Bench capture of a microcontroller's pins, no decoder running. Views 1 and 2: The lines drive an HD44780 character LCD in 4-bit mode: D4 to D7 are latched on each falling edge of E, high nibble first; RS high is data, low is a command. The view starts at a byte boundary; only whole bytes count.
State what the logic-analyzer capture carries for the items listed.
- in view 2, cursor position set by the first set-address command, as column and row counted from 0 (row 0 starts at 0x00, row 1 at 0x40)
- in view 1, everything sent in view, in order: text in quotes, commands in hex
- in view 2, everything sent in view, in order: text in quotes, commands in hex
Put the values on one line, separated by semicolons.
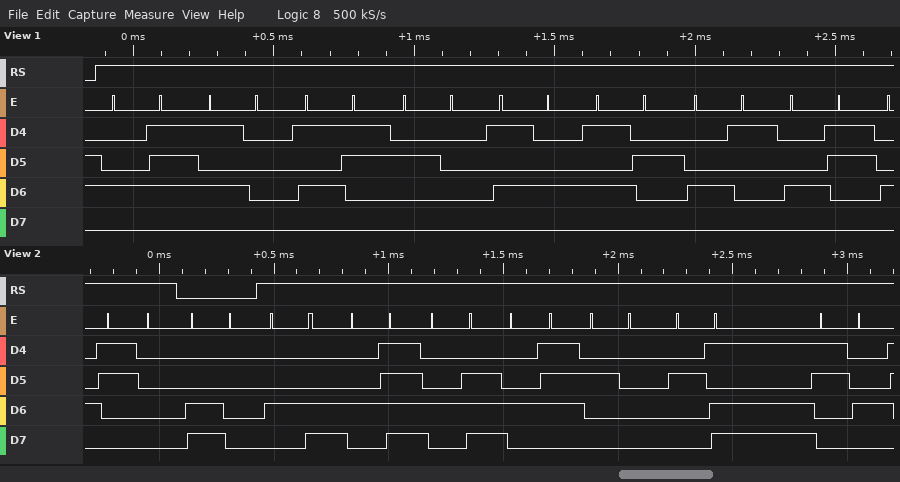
column 0, row 1; "GPS TRAC"; "0" 0xC0 "LONG -4"
